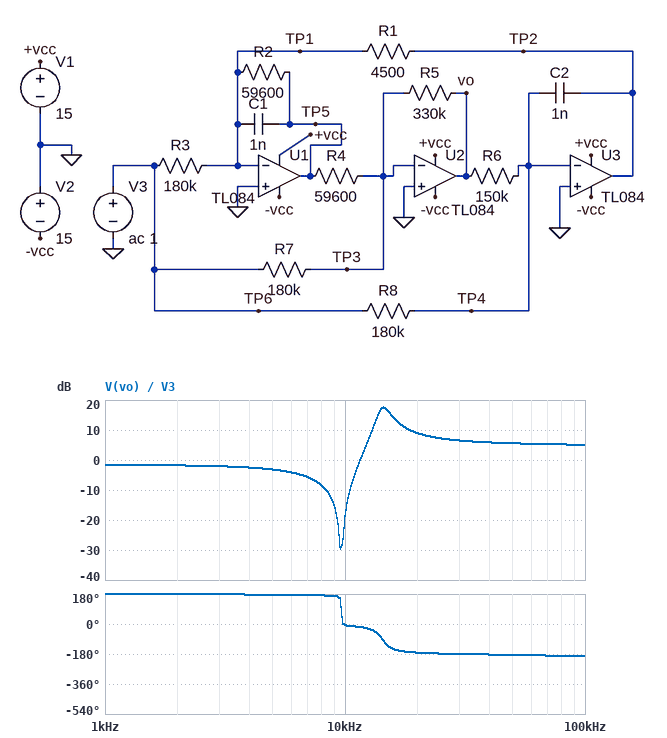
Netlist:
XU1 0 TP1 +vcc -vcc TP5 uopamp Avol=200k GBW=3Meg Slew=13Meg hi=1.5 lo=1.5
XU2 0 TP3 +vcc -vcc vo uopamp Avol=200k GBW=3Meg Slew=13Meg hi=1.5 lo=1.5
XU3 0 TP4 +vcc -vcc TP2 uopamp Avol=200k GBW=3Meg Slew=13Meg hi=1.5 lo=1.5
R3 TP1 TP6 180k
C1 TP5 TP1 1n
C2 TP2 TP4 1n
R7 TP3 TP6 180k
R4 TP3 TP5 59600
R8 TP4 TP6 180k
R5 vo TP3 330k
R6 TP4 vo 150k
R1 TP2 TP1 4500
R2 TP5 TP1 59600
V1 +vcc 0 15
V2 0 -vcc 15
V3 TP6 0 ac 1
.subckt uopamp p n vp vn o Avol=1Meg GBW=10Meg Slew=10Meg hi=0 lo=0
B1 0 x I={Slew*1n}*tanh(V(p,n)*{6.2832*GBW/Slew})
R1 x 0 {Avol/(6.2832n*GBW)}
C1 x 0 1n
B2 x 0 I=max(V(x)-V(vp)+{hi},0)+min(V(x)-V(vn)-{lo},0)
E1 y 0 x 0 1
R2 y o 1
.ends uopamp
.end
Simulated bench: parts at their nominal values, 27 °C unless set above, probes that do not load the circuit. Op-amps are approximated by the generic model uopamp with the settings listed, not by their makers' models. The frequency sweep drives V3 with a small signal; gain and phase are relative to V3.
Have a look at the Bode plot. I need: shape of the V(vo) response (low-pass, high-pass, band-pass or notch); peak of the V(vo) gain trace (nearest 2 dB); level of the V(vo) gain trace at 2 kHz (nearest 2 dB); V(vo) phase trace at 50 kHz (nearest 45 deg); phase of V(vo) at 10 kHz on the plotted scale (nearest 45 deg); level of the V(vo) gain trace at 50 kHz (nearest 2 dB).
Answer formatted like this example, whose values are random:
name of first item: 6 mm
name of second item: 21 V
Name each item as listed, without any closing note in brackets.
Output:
shape of the V(vo) response: band-pass
peak of the V(vo) gain trace: 18 dB
level of the V(vo) gain trace at 2 kHz: -2 dB
V(vo) phase trace at 50 kHz: -180 deg
phase of V(vo) at 10 kHz on the plotted scale: 0 deg
level of the V(vo) gain trace at 50 kHz: 6 dB
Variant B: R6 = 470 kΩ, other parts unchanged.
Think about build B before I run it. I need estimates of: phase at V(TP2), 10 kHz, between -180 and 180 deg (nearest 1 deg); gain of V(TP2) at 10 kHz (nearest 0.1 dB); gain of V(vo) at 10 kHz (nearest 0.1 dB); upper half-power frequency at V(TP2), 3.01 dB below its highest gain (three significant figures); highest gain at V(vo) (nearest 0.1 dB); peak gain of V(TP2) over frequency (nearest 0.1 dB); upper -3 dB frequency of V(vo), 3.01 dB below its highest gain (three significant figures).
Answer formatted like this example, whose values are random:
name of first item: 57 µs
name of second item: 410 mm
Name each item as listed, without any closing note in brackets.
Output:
phase at V(TP2), 10 kHz, between -180 and 180 deg: 85 deg
gain of V(TP2) at 10 kHz: -21.9 dB
gain of V(vo) at 10 kHz: -10.5 dB
upper half-power frequency at V(TP2), 3.01 dB below its highest gain: 9.19 kHz
highest gain at V(vo): 10.7 dB
peak gain of V(TP2) over frequency: -16.0 dB
upper -3 dB frequency of V(vo), 3.01 dB below its highest gain: 8.18 kHz
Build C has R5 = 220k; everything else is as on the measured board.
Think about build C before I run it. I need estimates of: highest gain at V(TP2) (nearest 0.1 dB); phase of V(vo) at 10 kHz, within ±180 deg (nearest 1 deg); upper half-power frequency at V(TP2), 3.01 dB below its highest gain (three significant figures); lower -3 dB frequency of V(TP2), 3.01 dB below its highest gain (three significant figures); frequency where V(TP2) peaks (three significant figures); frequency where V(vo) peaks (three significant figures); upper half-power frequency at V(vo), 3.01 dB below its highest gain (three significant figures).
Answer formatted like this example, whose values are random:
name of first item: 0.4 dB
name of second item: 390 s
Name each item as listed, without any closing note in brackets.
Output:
highest gain at V(TP2): -14.2 dB
phase of V(vo) at 10 kHz, within ±180 deg: -28 deg
upper half-power frequency at V(TP2), 3.01 dB below its highest gain: 12.8 kHz
lower -3 dB frequency of V(TP2), 3.01 dB below its highest gain: 10.6 kHz
frequency where V(TP2) peaks: 11.7 kHz
frequency where V(vo) peaks: 12.3 kHz
upper half-power frequency at V(vo), 3.01 dB below its highest gain: 16.1 kHz
